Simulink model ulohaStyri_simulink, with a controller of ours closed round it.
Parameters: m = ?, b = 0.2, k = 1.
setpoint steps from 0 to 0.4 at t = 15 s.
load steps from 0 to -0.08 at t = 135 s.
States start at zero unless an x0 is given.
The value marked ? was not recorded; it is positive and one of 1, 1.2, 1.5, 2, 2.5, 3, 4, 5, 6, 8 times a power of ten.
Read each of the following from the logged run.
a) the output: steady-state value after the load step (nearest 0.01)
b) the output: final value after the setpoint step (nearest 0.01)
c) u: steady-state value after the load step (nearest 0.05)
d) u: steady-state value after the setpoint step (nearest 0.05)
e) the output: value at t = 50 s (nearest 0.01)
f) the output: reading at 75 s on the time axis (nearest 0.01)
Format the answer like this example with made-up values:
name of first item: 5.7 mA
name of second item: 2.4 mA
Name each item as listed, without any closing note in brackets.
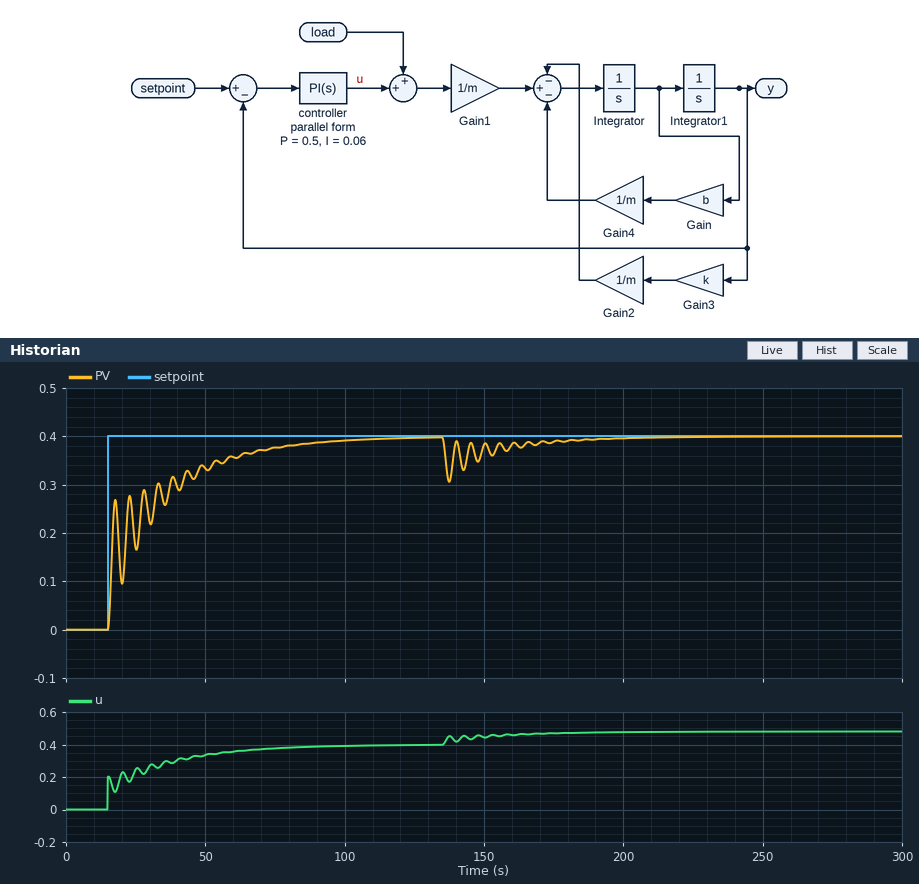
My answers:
the output: steady-state value after the load step: 0.40
the output: final value after the setpoint step: 0.40
u: steady-state value after the load step: 0.50
u: steady-state value after the setpoint step: 0.40
the output: value at t = 50 s: 0.33
the output: reading at 75 s on the time axis: 0.38
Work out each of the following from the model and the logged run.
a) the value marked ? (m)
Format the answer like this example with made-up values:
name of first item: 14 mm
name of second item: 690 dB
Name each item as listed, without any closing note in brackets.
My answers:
the value marked ?: 1
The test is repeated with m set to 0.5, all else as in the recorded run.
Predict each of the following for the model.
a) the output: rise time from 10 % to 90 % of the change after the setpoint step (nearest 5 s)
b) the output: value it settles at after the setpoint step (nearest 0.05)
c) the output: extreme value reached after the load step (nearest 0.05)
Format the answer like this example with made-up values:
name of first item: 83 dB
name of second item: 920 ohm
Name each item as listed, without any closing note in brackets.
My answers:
the output: rise time from 10 % to 90 % of the change after the setpoint step: 45 s
the output: value it settles at after the setpoint step: 0.40
the output: extreme value reached after the load step: 0.30
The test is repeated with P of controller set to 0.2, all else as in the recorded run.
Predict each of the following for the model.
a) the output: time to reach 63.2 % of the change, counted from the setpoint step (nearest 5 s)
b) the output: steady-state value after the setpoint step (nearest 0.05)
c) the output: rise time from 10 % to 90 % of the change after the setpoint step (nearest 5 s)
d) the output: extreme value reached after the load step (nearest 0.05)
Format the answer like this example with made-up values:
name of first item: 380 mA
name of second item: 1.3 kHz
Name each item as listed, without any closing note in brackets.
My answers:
the output: time to reach 63.2 % of the change, counted from the setpoint step: 15 s
the output: steady-state value after the setpoint step: 0.40
the output: rise time from 10 % to 90 % of the change after the setpoint step: 40 s
the output: extreme value reached after the load step: 0.30
